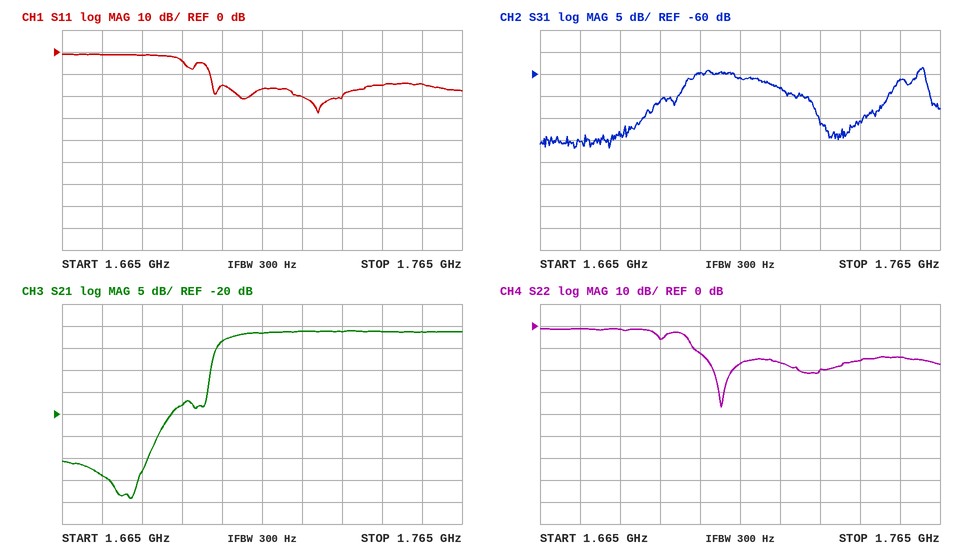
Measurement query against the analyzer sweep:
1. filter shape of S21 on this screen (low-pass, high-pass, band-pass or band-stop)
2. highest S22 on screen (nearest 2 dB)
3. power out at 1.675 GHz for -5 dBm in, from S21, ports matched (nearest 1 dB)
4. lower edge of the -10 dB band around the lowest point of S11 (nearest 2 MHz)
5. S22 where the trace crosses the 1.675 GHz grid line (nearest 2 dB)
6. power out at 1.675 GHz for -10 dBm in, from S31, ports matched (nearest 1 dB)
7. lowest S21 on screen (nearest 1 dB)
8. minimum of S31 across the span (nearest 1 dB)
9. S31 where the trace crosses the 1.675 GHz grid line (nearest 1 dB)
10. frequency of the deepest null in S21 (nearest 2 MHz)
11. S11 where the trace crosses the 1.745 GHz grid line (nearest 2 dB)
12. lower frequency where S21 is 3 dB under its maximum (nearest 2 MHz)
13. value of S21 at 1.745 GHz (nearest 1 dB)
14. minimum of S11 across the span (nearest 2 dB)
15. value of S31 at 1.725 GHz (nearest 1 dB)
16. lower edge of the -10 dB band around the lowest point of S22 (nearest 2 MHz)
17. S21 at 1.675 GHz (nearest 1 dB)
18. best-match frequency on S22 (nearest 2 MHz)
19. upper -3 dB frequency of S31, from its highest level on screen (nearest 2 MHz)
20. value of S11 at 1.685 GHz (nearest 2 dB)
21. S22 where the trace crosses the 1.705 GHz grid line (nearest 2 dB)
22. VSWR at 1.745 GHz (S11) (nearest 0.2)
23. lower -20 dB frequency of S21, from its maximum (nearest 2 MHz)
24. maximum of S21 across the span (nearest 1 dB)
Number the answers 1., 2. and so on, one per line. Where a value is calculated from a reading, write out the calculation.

1. high-pass
2. -2 dB
3. -5 dBm + (-34 dB) = -39 dBm
4. 1.702 GHz
5. -2 dB
6. -10 dBm + (-75 dB) = -85 dBm
7. -39 dB
8. -77 dB
9. -75 dB
10. 1.682 GHz
11. -16 dB
12. 1.704 GHz
13. -1 dB
14. -28 dB
15. -63 dB
16. 1.704 GHz
17. -34 dB
18. 1.710 GHz
19. 1.762 GHz
20. -2 dB
21. -12 dB
22. |Γ| = 10^(-16/20) = 0.1585; VSWR = (1 + 0.1585)/(1 − 0.1585) ≈ 1.4
23. 1.692 GHz
24. -1 dB
